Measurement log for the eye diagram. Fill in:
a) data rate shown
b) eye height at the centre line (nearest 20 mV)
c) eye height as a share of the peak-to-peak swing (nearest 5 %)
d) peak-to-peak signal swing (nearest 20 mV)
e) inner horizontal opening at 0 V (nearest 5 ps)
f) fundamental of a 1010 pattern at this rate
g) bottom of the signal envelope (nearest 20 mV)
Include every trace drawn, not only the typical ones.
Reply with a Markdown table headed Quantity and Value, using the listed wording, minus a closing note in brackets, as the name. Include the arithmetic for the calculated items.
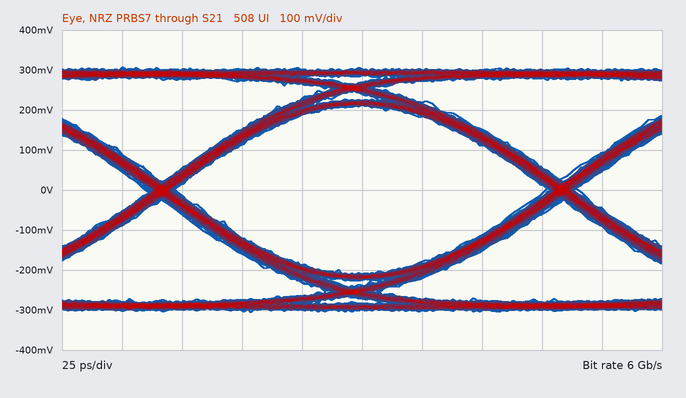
| Quantity | Value |
|---|---|
| data rate shown | 6 Gb/s |
| eye height at the centre line | 420 mV |
| eye height as a share of the peak-to-peak swing | 420 mV / 620 mV ≈ 67.7 %, so 70 % to the nearest 5 % |
| peak-to-peak signal swing | 620 mV |
| inner horizontal opening at 0 V | 155 ps |
| fundamental of a 1010 pattern at this rate | 3 GHz |
| bottom of the signal envelope | -300 mV |
